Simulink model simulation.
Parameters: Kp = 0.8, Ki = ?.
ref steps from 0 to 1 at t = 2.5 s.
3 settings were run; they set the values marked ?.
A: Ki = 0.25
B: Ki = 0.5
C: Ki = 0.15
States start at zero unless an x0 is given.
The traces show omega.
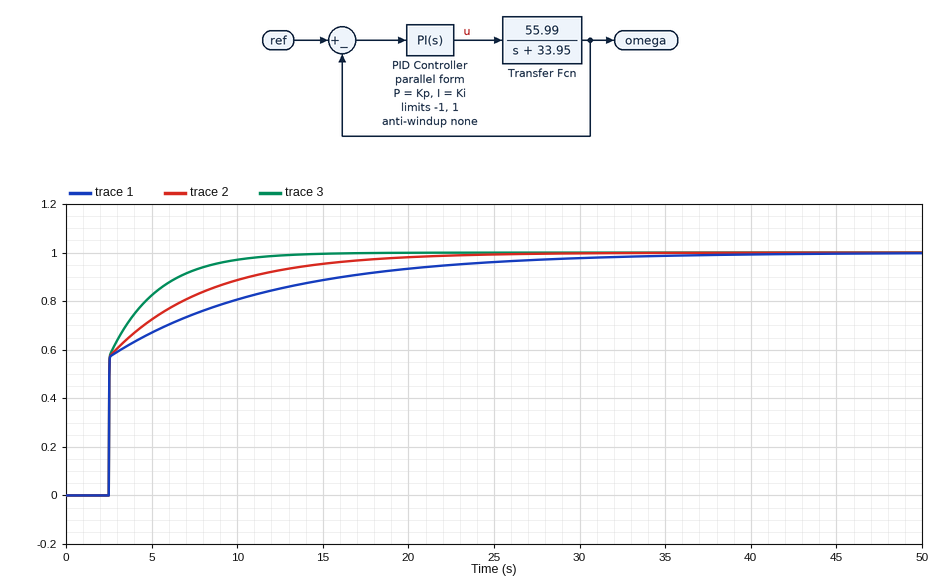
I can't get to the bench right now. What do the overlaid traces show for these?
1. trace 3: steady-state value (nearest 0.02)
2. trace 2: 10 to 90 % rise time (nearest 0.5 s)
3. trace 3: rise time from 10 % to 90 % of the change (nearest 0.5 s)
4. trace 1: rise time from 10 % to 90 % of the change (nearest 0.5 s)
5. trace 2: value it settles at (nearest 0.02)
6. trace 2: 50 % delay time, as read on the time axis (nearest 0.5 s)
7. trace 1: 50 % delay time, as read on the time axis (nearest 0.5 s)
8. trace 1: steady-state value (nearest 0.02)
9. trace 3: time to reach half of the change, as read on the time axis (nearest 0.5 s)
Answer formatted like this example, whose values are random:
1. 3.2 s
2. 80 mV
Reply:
1. 1.00
2. 8.0 s
3. 4.0 s
4. 13.5 s
5. 1.00
6. 2.5 s
7. 2.5 s
8. 1.00
9. 2.5 s
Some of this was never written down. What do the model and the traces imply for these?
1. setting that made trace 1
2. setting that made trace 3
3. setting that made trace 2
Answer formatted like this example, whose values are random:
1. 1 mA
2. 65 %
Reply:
1. C
2. B
3. A
